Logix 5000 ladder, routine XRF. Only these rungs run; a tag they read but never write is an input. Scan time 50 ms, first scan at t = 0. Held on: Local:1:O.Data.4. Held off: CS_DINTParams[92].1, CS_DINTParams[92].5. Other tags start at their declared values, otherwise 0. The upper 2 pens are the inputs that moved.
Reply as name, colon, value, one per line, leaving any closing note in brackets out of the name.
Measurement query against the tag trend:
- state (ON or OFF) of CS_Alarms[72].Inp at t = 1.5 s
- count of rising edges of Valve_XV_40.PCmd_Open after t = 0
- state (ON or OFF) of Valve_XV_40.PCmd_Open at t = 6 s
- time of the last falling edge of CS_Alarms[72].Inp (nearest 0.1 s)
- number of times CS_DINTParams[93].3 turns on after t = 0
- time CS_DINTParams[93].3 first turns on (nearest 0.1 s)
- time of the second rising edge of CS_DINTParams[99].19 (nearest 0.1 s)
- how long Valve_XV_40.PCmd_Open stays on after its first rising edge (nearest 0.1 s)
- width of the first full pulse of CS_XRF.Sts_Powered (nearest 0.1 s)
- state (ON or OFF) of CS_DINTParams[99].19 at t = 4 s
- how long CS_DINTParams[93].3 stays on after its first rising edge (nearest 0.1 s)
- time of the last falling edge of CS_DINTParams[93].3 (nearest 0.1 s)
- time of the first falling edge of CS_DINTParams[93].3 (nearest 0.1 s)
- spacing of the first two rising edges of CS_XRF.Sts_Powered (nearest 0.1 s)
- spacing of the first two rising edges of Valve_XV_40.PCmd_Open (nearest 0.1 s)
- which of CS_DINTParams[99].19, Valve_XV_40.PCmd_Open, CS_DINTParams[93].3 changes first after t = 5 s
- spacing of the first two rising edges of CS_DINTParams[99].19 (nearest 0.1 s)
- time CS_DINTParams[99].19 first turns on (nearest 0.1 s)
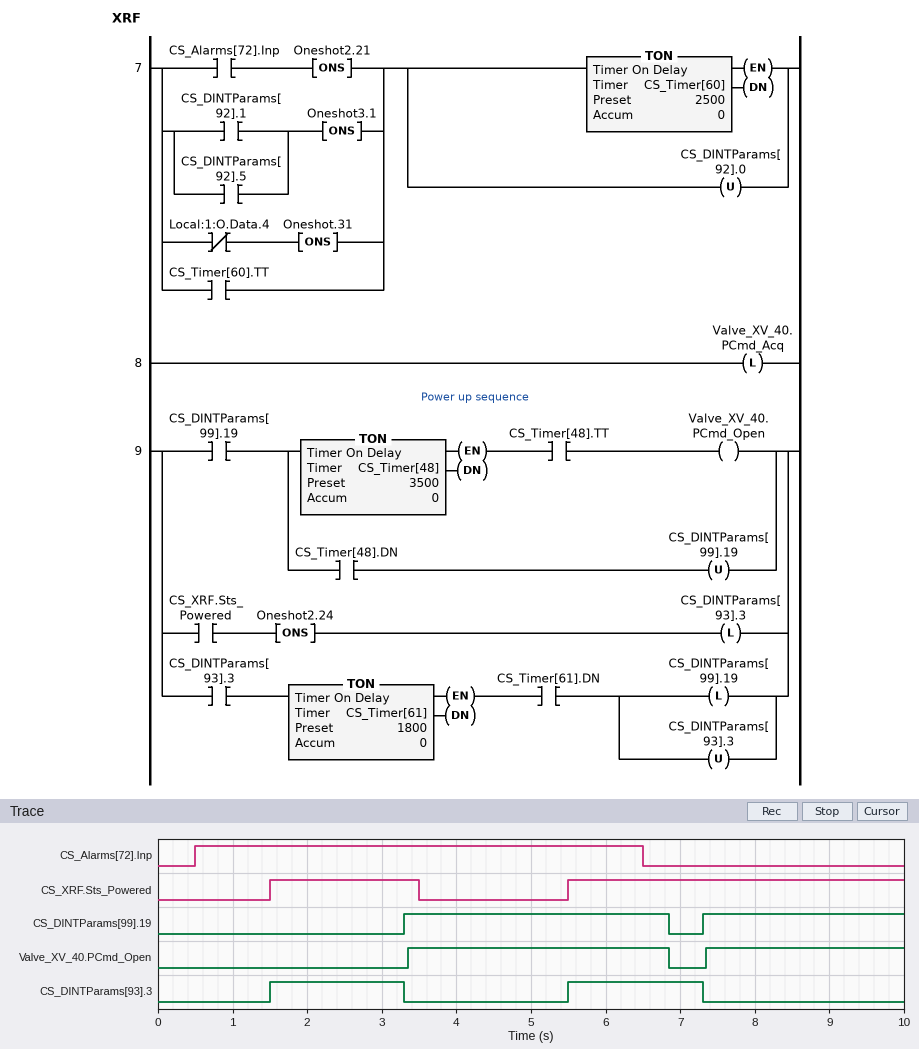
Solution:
state (ON or OFF) of CS_Alarms[72].Inp at t = 1.5 s: ON
count of rising edges of Valve_XV_40.PCmd_Open after t = 0: 2
state (ON or OFF) of Valve_XV_40.PCmd_Open at t = 6 s: ON
time of the last falling edge of CS_Alarms[72].Inp: 6.5 s
number of times CS_DINTParams[93].3 turns on after t = 0: 2
time CS_DINTParams[93].3 first turns on: 1.5 s
time of the second rising edge of CS_DINTParams[99].19: 7.3 s
how long Valve_XV_40.PCmd_Open stays on after its first rising edge: 3.5 s
width of the first full pulse of CS_XRF.Sts_Powered: 2.0 s
state (ON or OFF) of CS_DINTParams[99].19 at t = 4 s: ON
how long CS_DINTParams[93].3 stays on after its first rising edge: 1.8 s
time of the last falling edge of CS_DINTParams[93].3: 7.3 s
time of the first falling edge of CS_DINTParams[93].3: 3.3 s
spacing of the first two rising edges of CS_XRF.Sts_Powered: 4.0 s
spacing of the first two rising edges of Valve_XV_40.PCmd_Open: 4.0 s
which of CS_DINTParams[99].19, Valve_XV_40.PCmd_Open, CS_DINTParams[93].3 changes first after t = 5 s: CS_DINTParams[93].3
spacing of the first two rising edges of CS_DINTParams[99].19: 4.0 s
time CS_DINTParams[99].19 first turns on: 3.3 s
